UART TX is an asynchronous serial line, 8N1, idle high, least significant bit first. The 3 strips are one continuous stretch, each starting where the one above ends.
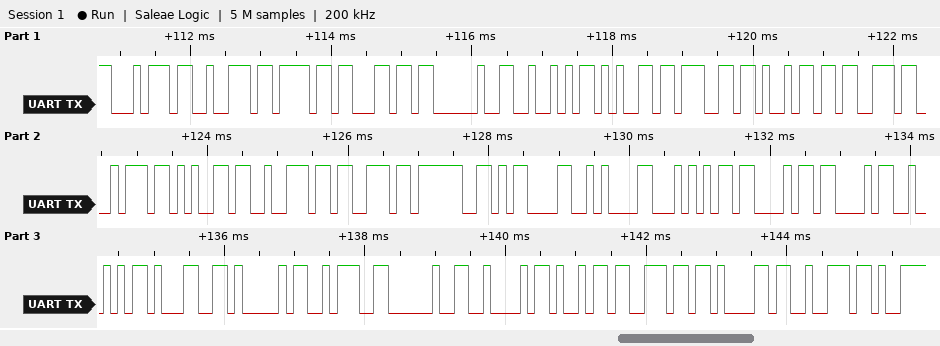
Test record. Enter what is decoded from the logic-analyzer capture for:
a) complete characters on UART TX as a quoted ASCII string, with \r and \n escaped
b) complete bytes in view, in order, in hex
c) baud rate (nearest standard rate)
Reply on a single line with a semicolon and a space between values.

"trol Registers?\r\nTCCR1A: Binar"; 74 72 6F 6C 20 52 65 67 69 73 74 65 72 73 3F 0D 0A 54 43 43 52 31 41 3A 20 42 69 6E 61 72; 9600 baud
